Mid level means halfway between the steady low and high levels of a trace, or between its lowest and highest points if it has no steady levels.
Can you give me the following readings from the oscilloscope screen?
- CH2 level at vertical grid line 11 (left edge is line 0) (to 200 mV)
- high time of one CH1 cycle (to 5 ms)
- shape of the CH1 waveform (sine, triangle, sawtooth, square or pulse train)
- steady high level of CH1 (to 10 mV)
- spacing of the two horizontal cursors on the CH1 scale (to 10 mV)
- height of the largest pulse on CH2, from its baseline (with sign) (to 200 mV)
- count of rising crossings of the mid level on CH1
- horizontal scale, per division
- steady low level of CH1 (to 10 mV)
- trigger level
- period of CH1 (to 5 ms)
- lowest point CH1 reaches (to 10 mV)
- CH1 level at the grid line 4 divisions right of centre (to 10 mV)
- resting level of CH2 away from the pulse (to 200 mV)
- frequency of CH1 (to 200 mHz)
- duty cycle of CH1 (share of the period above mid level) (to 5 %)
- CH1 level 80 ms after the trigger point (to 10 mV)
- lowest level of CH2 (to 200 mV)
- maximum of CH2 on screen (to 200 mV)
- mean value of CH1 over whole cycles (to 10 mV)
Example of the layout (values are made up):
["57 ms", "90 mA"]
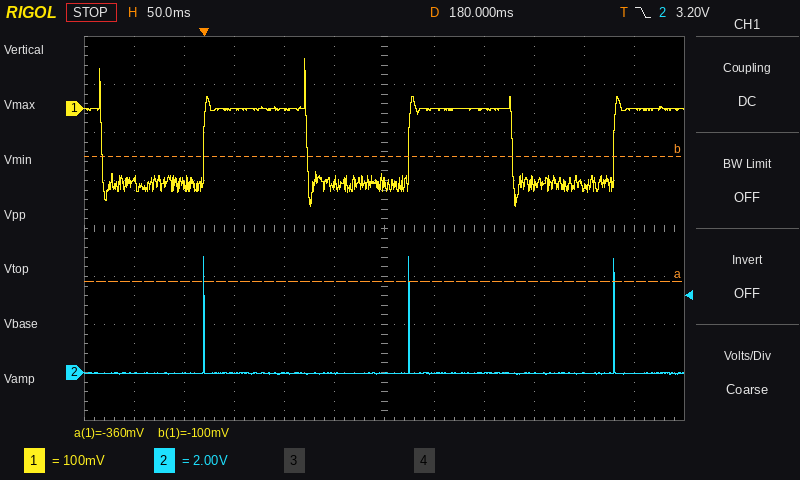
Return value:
["0.0 V", "105 ms", "square", "0 mV", "260 mV", "+4.8 V", "3", "50 ms", "-150 mV", "3.20 V", "205 ms", "-200 mV", "-160 mV", "0.0 V", "4.8 Hz", "50 %", "0 mV", "0.0 V", "4.8 V", "-80 mV"]
